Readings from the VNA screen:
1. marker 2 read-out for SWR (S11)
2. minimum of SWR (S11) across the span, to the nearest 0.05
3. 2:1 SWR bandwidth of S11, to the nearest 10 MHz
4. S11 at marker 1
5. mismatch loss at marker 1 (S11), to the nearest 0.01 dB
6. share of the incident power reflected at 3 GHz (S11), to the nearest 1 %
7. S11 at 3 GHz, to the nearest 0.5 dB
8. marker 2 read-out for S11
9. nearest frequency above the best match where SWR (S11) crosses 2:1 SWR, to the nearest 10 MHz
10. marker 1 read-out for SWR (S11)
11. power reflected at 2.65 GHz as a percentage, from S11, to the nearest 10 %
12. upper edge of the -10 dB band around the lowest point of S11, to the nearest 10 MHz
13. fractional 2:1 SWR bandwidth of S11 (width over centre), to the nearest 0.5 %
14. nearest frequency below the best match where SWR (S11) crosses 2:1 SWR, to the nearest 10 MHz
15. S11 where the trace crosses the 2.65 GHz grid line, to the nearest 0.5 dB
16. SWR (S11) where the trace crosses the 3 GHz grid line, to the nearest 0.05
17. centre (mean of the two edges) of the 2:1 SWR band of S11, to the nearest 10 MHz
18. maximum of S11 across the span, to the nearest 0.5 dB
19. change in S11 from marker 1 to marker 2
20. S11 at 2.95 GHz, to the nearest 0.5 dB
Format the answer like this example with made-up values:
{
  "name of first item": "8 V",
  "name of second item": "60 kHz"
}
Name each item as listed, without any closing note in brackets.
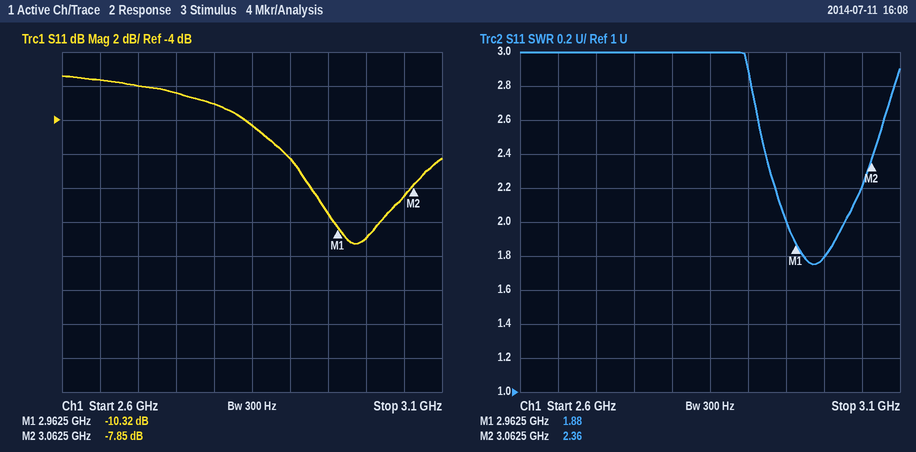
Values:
{
  "marker 2 read-out for SWR": "2.36",
  "minimum of SWR (S11) across the span, to the nearest 0.05": "1.75",
  "2:1 SWR bandwidth of S11, to the nearest 10 MHz": "80 MHz",
  "S11 at marker 1": "-10.32 dB",
  "mismatch loss at marker 1 (S11), to the nearest 0.01 dB": "0.42 dB",
  "share of the incident power reflected at 3 GHz (S11), to the nearest 1 %": "8 %",
  "S11 at 3 GHz, to the nearest 0.5 dB": "-11.0 dB",
  "marker 2 read-out for S11": "-7.85 dB",
  "nearest frequency above the best match where SWR (S11) crosses 2:1 SWR, to the nearest 10 MHz": "3.03 GHz",
  "marker 1 read-out for SWR": "1.88",
  "power reflected at 2.65 GHz as a percentage, from S11, to the nearest 10 %": "70 %",
  "upper edge of the -10 dB band around the lowest point of S11, to the nearest 10 MHz": "3.02 GHz",
  "fractional 2:1 SWR bandwidth of S11 (width over centre), to the nearest 0.5 %": "2.5 %",
  "nearest frequency below the best match where SWR (S11) crosses 2:1 SWR, to the nearest 10 MHz": "2.95 GHz",
  "S11 where the trace crosses the 2.65 GHz grid line, to the nearest 0.5 dB": "-1.5 dB",
  "SWR (S11) where the trace crosses the 3 GHz grid line, to the nearest 0.05": "1.80",
  "centre (mean of the two edges) of the 2:1 SWR band of S11, to the nearest 10 MHz": "2.99 GHz",
  "maximum of S11 across the span, to the nearest 0.5 dB": "-1.5 dB",
  "change in S11 from marker 1 to marker 2": "2.47 dB",
  "S11 at 2.95 GHz, to the nearest 0.5 dB": "-9.5 dB"
}
